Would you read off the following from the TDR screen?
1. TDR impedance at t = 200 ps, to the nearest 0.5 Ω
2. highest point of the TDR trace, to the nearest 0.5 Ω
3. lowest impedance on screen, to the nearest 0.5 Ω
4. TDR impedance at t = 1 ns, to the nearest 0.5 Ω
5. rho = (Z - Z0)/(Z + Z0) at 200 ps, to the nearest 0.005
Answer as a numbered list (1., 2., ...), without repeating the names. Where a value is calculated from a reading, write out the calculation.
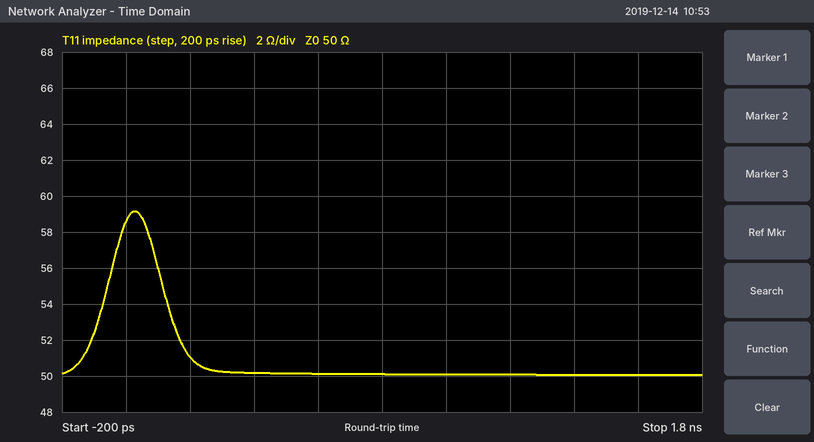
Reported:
1. 51.0 Ω
2. 59.0 Ω
3. 50.0 Ω
4. 50.0 Ω
5. (51 − 50)/(51 + 50) ≈ +0.010
